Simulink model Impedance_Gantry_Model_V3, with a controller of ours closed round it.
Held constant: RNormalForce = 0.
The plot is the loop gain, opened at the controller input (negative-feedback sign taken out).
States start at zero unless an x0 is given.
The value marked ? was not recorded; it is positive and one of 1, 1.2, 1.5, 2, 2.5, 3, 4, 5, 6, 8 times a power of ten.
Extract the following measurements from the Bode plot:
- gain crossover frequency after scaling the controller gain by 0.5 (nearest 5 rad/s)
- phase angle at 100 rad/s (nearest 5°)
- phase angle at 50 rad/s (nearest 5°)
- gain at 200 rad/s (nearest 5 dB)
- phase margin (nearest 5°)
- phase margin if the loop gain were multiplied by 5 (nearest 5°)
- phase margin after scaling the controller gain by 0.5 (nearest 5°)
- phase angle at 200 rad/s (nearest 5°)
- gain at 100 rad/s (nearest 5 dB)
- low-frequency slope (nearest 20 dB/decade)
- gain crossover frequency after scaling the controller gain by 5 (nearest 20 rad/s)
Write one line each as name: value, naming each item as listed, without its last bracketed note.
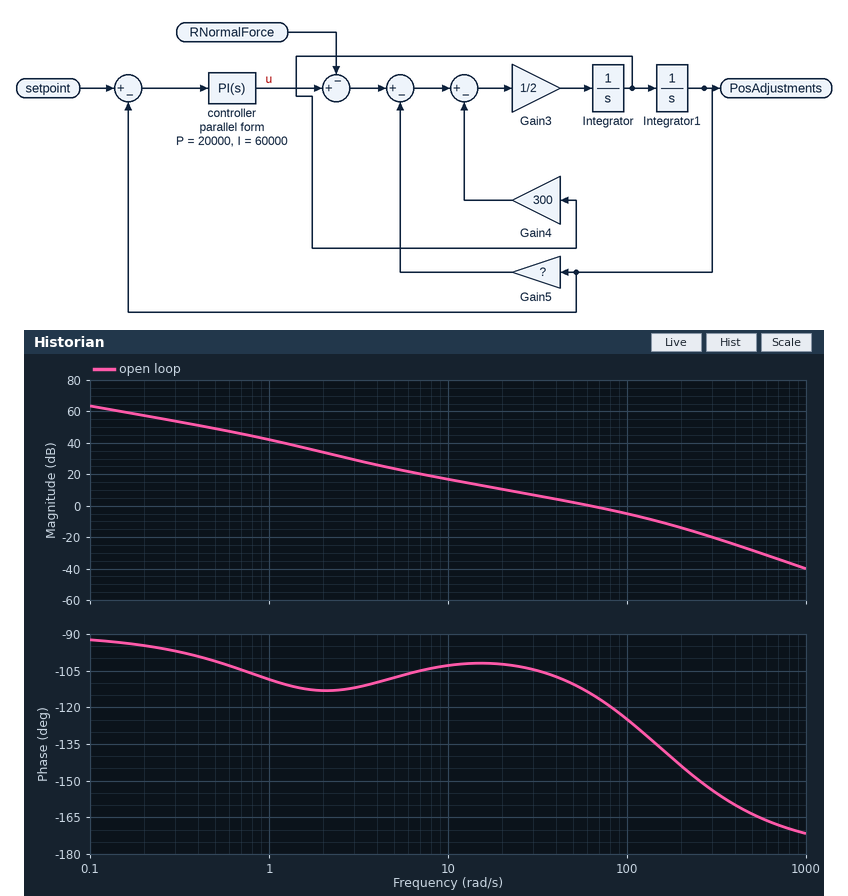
gain crossover frequency after scaling the controller gain by 0.5: 35 rad/s
phase angle at 100 rad/s: -125°
phase angle at 50 rad/s: -110°
gain at 200 rad/s: -15 dB
phase margin: 65°
phase margin if the loop gain were multiplied by 5: 35°
phase margin after scaling the controller gain by 0.5: 75°
phase angle at 200 rad/s: -145°
gain at 100 rad/s: -5 dB
low-frequency slope: -20 dB/decade
gain crossover frequency after scaling the controller gain by 5: 200 rad/s
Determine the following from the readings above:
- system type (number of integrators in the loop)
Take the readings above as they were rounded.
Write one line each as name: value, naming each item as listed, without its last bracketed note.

system type: 1
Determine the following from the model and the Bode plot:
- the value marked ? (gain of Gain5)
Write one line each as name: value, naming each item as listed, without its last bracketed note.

the value marked ?: 400
